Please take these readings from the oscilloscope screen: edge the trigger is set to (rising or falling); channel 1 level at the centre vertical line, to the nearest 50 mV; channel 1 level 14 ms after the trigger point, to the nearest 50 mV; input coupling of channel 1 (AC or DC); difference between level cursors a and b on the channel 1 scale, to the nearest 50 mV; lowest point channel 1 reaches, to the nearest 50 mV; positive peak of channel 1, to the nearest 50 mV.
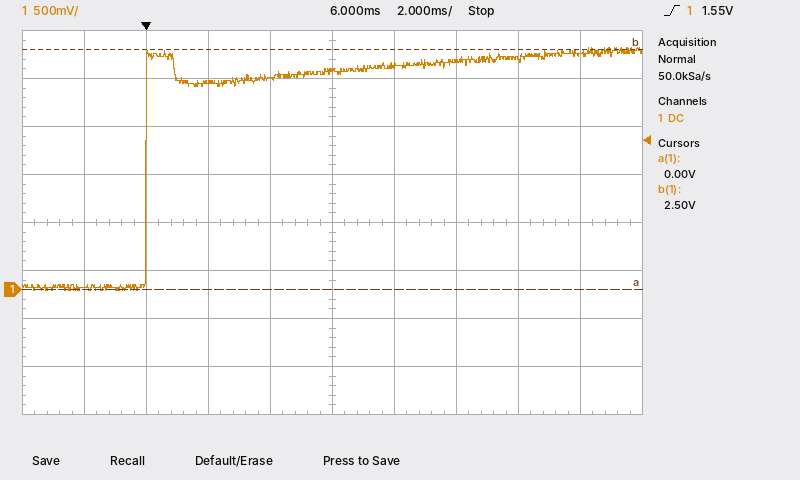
rising
2.25 V
2.45 V
DC
2.50 V
0 mV
2.50 V
